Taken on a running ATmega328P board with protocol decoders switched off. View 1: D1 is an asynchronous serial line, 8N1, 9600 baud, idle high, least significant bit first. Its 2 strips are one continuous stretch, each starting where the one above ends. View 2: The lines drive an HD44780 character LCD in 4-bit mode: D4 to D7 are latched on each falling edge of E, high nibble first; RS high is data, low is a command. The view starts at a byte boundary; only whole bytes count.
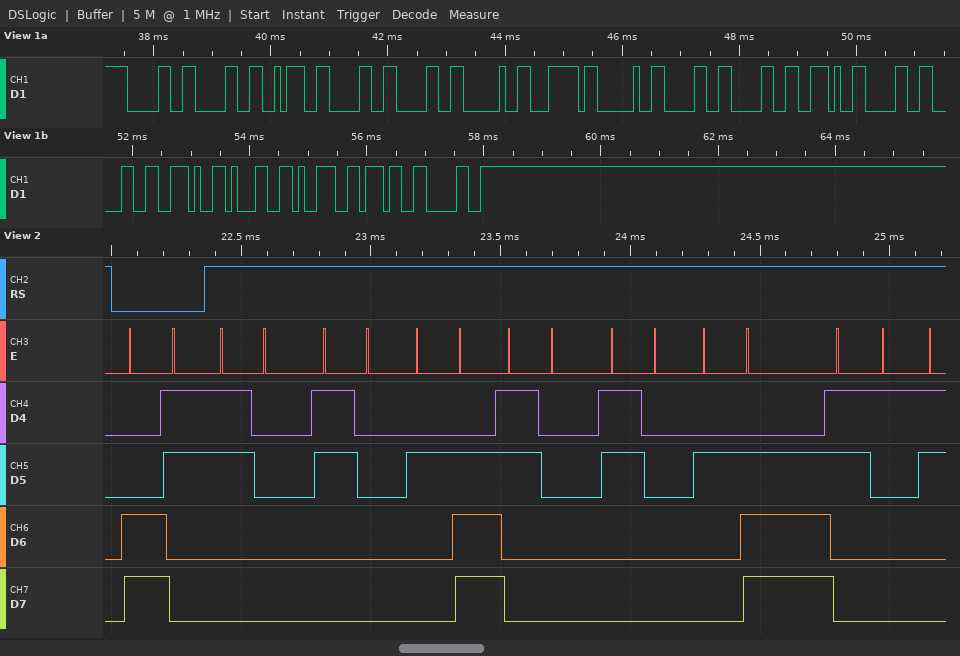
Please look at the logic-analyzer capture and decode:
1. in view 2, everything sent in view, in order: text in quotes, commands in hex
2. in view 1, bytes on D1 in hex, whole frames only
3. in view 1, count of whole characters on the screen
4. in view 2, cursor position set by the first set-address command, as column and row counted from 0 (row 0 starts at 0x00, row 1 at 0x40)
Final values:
0xC3 "00.00.1"
30 30 3A 30 30 20 7C 20 30 30 2E 30 30 2E 31 39 37 30
18
column 3, row 1
